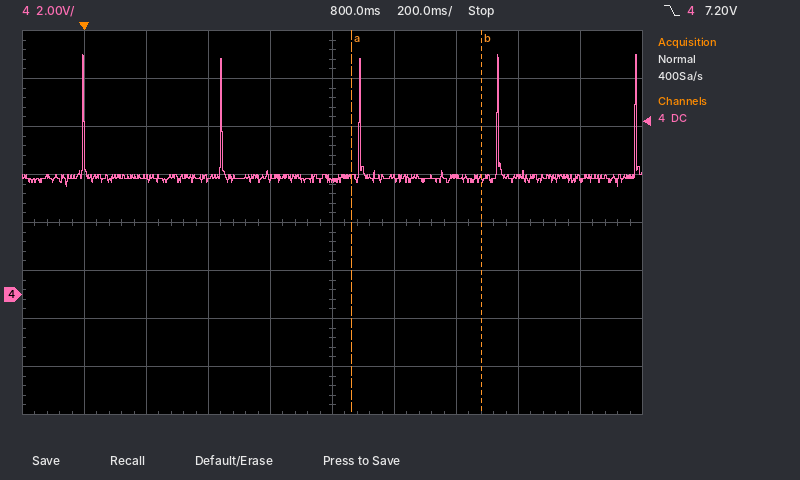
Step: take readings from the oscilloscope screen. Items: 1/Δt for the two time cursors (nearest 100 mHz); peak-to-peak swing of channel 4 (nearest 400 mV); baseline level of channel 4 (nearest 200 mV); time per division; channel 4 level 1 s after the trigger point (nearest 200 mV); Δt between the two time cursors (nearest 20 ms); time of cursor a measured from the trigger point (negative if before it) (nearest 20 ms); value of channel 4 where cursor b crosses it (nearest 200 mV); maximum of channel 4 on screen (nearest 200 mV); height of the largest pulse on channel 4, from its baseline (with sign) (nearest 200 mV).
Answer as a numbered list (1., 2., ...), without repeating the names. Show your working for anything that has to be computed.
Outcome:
1. 1 / 420 ms ≈ 2.4 Hz
2. 5.6 V
3. 4.8 V
4. 200 ms
5. 4.8 V
6. 420 ms
7. +860 ms
8. 4.8 V
9. 10.0 V
10. 10.0 V − (4.8 V) = +5.2 V
